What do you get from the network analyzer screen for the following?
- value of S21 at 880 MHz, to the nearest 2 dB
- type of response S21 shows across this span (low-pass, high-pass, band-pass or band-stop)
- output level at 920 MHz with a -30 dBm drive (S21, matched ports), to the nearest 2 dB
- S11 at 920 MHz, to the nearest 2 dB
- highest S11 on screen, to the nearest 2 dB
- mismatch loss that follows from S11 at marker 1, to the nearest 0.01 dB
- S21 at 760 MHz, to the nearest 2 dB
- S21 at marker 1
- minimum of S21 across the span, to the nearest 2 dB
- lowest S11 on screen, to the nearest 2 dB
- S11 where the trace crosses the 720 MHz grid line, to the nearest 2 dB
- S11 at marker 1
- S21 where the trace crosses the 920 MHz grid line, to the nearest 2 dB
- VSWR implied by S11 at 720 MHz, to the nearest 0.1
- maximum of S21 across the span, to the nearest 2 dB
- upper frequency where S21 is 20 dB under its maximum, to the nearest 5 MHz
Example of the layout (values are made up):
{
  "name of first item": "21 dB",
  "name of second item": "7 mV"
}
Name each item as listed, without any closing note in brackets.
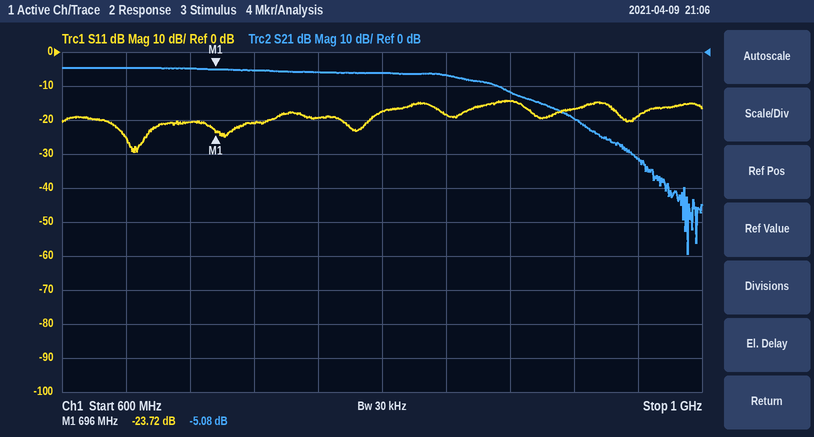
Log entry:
{
  "value of S21 at 880 MHz, to the nearest 2 dB": "-12 dB",
  "type of response S21 shows across this span": "low-pass",
  "output level at 920 MHz with a -30 dBm drive (S21, matched ports), to the nearest 2 dB": "-50 dBm",
  "S11 at 920 MHz, to the nearest 2 dB": "-16 dB",
  "highest S11 on screen, to the nearest 2 dB": "-14 dB",
  "mismatch loss that follows from S11 at marker 1, to the nearest 0.01 dB": "0.02 dB",
  "S21 at 760 MHz, to the nearest 2 dB": "-6 dB",
  "S21 at marker 1": "-5.08 dB",
  "minimum of S21 across the span, to the nearest 2 dB": "-60 dB",
  "lowest S11 on screen, to the nearest 2 dB": "-30 dB",
  "S11 where the trace crosses the 720 MHz grid line, to the nearest 2 dB": "-20 dB",
  "S11 at marker 1": "-23.72 dB",
  "S21 where the trace crosses the 920 MHz grid line, to the nearest 2 dB": "-20 dB",
  "VSWR implied by S11 at 720 MHz, to the nearest 0.1": "1.2",
  "maximum of S21 across the span, to the nearest 2 dB": "-4 dB",
  "upper frequency where S21 is 20 dB under its maximum, to the nearest 5 MHz": "935 MHz"
}
